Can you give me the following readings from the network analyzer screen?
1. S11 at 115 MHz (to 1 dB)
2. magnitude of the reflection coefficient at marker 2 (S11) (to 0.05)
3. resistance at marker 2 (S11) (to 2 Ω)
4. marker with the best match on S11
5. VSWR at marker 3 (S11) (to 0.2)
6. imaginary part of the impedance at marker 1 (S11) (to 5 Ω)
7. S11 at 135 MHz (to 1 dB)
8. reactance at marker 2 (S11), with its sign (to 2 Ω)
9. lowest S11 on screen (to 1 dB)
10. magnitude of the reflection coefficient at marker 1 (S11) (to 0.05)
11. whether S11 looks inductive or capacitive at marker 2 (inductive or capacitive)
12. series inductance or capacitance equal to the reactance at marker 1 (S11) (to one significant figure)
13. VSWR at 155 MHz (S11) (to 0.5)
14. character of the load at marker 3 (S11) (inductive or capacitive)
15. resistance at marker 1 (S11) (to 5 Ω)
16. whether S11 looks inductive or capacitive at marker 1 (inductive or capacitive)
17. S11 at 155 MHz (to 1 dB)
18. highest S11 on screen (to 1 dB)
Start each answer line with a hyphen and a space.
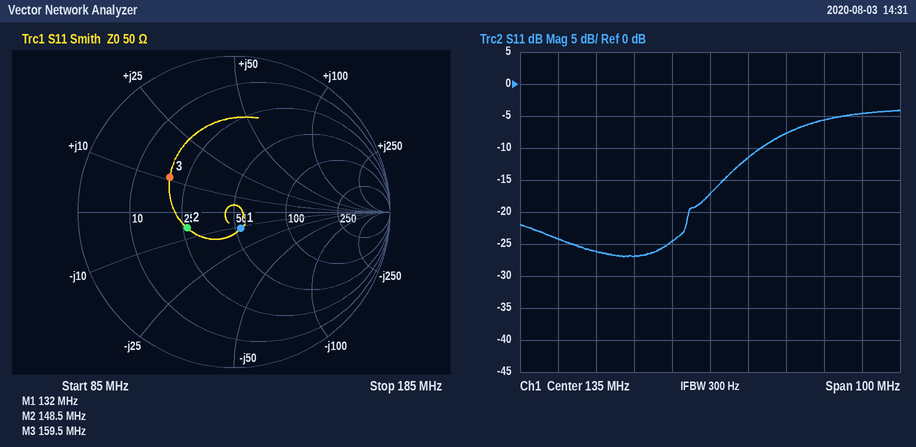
- -27 dB
- 0.30
- 26 Ω
- marker 1
- 2.8
- -10 Ω
- -17 dB
- -6 Ω
- -27 dB
- 0.10
- capacitive
- 100 pF
- 2.5
- inductive
- 55 Ω
- capacitive
- -8 dB
- -4 dB
